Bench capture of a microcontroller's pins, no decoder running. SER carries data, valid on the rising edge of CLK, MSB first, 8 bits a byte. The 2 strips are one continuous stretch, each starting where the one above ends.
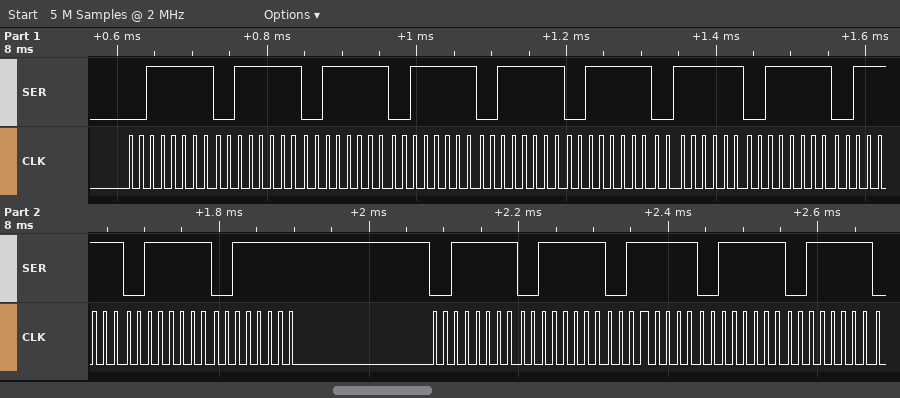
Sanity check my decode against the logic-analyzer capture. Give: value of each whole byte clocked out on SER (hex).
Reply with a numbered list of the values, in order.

1. 3F 3F 3F 3F 3F 3F 3F 3F 3F 3F 3F 3F 3F 3F 3F 3F
